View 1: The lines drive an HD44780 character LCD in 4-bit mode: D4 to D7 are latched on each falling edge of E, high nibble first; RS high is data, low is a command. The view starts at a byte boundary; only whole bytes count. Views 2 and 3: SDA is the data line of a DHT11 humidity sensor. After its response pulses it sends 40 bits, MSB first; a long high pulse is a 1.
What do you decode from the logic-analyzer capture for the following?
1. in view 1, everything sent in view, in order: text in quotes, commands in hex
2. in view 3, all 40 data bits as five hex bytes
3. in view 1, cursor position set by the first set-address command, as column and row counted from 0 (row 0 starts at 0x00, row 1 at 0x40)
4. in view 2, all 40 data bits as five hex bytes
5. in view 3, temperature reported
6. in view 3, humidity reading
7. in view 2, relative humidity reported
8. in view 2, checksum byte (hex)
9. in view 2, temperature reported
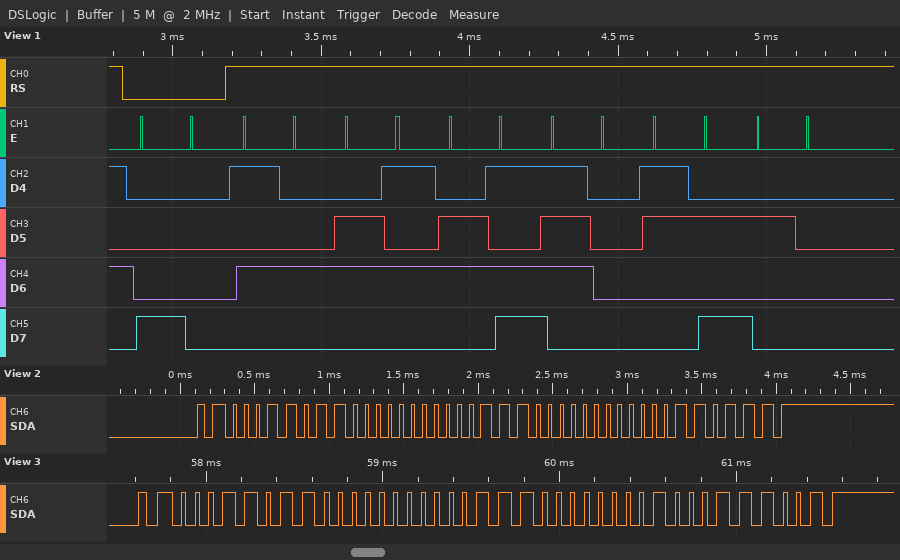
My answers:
0x80 "Temp: "
1B 00 1C 02 39
column 0, row 0
1B 00 1C 00 37
28.2 °C
27 %
27 %
0x37
28.0 °C
